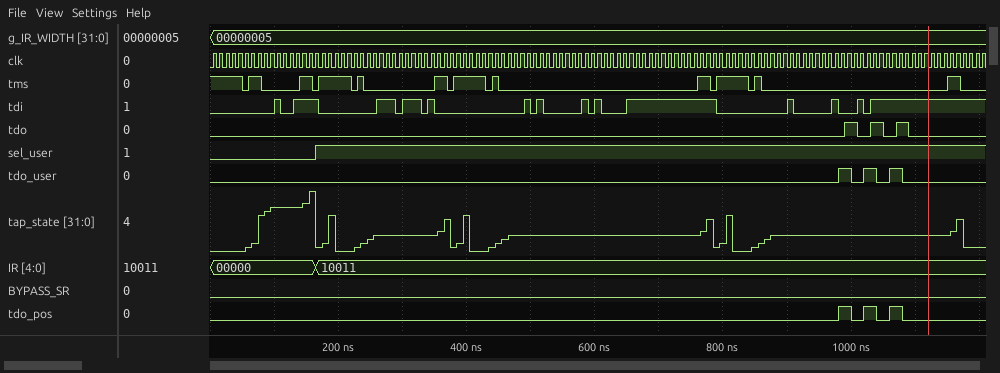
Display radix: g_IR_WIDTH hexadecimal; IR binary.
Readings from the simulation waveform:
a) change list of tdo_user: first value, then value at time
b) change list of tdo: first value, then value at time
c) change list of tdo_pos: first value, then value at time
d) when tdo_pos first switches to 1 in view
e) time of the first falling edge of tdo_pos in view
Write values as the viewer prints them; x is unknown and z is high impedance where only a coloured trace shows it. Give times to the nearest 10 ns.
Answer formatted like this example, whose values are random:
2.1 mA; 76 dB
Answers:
0, 1 at 980 ns, 0 at 1000 ns, 1 at 1020 ns, 0 at 1040 ns, 1 at 1060 ns, 0 at 1080 ns; 0, 1 at 990 ns, 0 at 1010 ns, 1 at 1030 ns, 0 at 1050 ns, 1 at 1070 ns, 0 at 1090 ns; 0, 1 at 980 ns, 0 at 1000 ns, 1 at 1020 ns, 0 at 1040 ns, 1 at 1060 ns, 0 at 1080 ns; 980 ns; 1000 ns
